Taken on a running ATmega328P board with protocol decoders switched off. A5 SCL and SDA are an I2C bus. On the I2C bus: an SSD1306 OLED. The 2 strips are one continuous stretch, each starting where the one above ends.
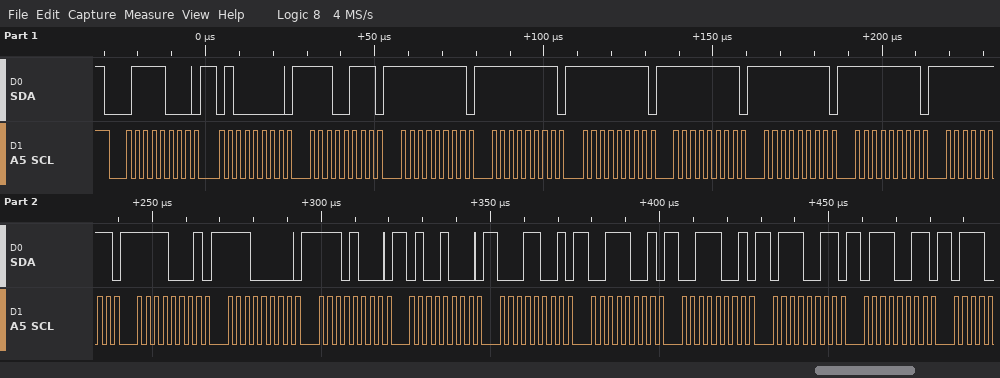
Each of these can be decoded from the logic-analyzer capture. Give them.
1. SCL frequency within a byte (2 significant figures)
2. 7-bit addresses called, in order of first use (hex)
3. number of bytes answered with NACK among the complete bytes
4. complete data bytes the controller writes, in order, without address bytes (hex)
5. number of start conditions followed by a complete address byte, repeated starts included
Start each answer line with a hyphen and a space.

- 400 kHz
- 0x3C
- 0
- 40 E7 FF FF FF FF FF FF FF F1 E0 E8 48 19 39 39 73 73
- 1
